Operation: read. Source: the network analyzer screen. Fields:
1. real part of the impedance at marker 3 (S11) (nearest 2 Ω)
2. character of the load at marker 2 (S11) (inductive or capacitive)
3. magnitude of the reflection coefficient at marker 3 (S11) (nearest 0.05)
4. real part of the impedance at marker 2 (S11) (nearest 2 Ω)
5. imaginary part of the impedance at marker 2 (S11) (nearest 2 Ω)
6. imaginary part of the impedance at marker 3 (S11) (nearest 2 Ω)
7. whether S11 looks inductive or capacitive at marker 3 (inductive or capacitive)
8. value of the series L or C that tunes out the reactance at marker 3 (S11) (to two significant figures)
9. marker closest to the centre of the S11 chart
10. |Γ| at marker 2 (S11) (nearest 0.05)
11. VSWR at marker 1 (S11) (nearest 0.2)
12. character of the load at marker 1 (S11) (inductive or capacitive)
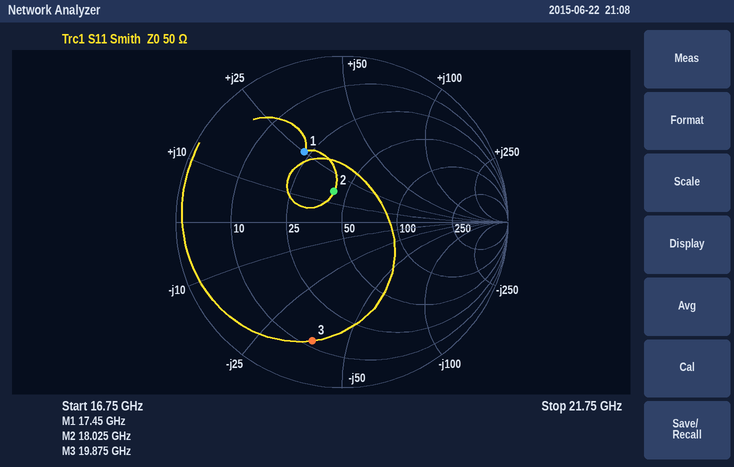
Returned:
12 Ω
inductive
0.75
42 Ω
+16 Ω
-38 Ω
capacitive
300 pH
marker 2
0.20
2.8
inductive
